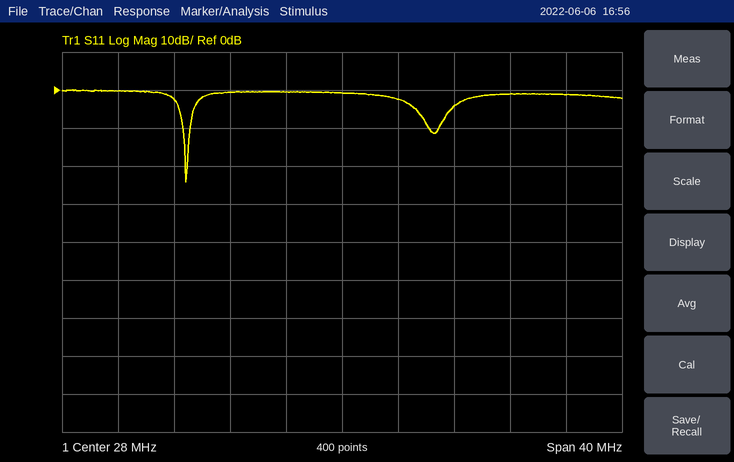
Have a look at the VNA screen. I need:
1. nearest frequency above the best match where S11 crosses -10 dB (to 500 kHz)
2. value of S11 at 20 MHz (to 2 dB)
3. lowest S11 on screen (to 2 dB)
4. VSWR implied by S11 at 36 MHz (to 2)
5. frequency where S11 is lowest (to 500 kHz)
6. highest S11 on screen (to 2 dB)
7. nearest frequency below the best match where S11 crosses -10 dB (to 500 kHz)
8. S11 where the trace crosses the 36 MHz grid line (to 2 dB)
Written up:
17.0 MHz
0 dB
-24 dB
4
17.0 MHz
0 dB
16.5 MHz
-4 dB
